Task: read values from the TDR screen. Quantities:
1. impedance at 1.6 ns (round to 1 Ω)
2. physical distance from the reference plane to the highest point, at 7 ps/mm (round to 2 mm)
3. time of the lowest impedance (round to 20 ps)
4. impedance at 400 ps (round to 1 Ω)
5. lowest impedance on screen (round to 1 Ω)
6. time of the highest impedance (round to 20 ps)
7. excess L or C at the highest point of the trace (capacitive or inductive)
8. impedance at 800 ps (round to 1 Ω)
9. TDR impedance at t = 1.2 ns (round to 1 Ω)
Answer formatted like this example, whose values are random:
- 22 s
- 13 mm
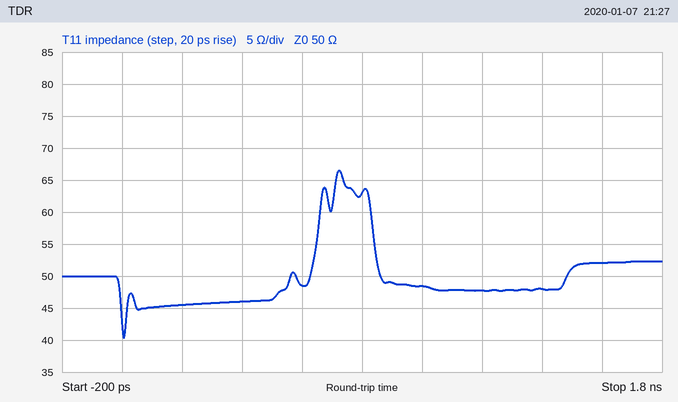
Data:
- 52 Ω
- 52 mm
- 0 ps
- 46 Ω
- 40 Ω
- 720 ps
- inductive
- 63 Ω
- 48 Ω
